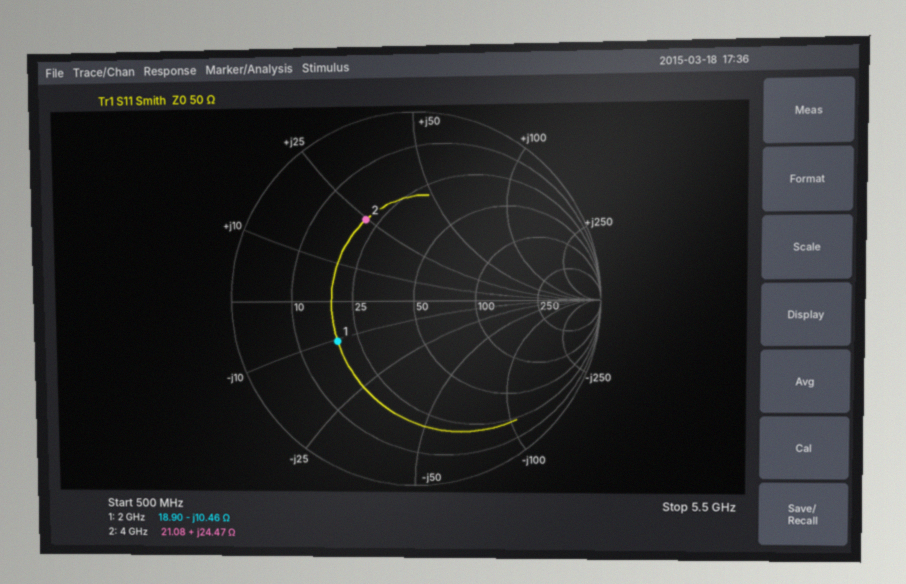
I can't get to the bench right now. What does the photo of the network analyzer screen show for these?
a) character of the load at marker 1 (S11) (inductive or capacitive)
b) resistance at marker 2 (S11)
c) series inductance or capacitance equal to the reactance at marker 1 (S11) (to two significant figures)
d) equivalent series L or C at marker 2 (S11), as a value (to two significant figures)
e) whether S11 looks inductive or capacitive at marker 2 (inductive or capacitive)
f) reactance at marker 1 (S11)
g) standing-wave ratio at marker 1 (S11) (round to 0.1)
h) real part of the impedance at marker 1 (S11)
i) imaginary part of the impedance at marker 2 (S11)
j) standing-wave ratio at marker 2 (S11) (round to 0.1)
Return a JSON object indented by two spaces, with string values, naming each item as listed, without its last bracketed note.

{
  "character of the load at marker 1 (S11)": "capacitive",
  "resistance at marker 2": "21.08 Ω",
  "series inductance or capacitance equal to the reactance at marker 1 (S11)": "7.6 pF",
  "equivalent series L or C at marker 2 (S11), as a value": "970 pH",
  "whether S11 looks inductive or capacitive at marker 2": "inductive",
  "reactance at marker 1": "-10.46 Ω",
  "standing-wave ratio at marker 1 (S11)": "2.8",
  "real part of the impedance at marker 1": "18.90 Ω",
  "imaginary part of the impedance at marker 2": "+24.47 Ω",
  "standing-wave ratio at marker 2 (S11)": "3.0"
}
